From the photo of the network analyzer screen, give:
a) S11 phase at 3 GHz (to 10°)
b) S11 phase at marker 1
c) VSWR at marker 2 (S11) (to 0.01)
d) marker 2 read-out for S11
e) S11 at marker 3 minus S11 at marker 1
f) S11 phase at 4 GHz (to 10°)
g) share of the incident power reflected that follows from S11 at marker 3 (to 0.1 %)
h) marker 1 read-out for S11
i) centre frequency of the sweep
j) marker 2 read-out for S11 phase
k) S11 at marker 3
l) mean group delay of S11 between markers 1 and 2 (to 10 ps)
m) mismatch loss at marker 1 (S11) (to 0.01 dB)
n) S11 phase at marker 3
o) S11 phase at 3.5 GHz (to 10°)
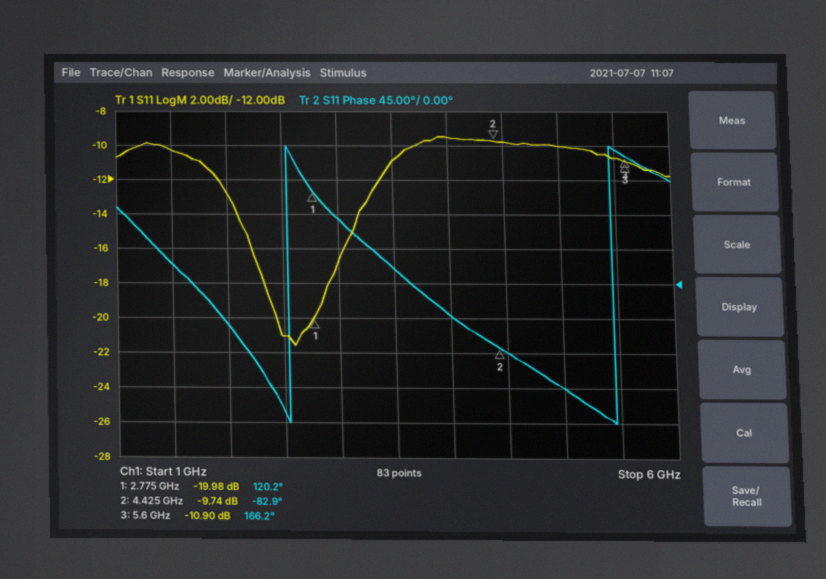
80°
120.2°
1.97
-9.74 dB
9.08 dB
-40°
8.1 %
-19.98 dB
3.5 GHz
-82.9°
-10.90 dB
340 ps
0.04 dB
166.2°
20°
